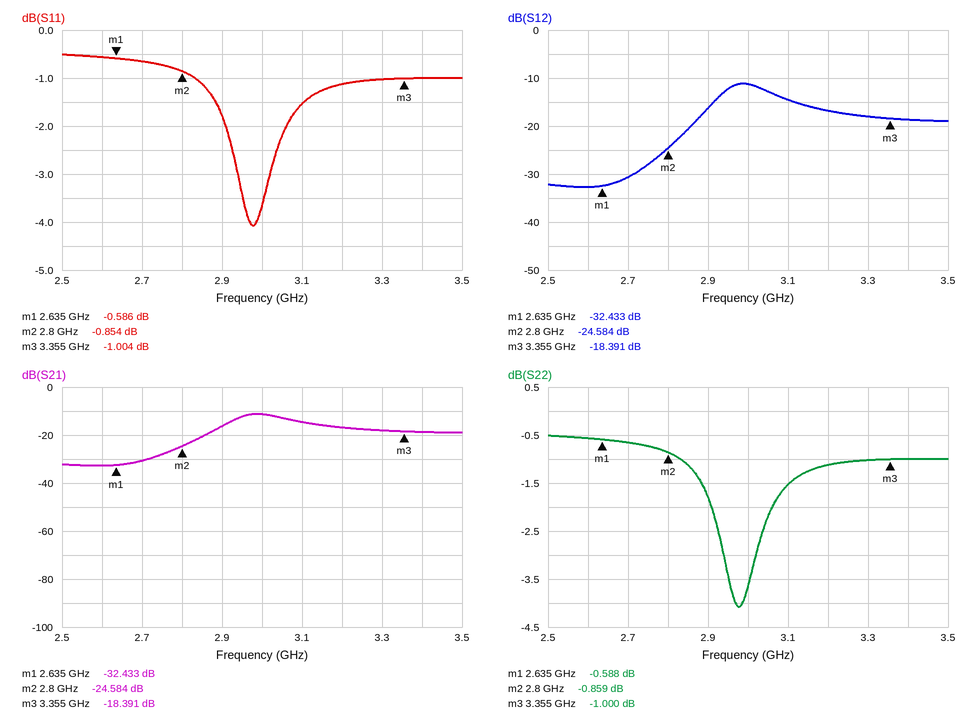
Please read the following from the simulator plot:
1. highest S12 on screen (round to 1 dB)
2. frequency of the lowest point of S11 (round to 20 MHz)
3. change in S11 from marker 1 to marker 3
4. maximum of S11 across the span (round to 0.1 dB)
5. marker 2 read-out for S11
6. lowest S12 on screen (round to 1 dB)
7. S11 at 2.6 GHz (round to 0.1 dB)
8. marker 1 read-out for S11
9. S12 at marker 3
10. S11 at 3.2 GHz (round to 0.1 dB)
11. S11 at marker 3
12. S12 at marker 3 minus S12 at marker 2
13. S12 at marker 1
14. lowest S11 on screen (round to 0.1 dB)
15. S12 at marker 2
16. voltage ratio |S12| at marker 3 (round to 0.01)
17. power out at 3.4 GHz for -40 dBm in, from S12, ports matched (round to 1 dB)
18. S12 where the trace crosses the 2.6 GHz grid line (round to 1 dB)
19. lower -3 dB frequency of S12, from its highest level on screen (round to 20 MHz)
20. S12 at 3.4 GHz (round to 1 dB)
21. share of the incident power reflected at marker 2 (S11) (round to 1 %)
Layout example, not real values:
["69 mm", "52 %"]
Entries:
["-11 dB", "2.98 GHz", "-0.418 dB", "-0.5 dB", "-0.854 dB", "-33 dB", "-0.6 dB", "-0.586 dB", "-18.391 dB", "-1.1 dB", "-1.004 dB", "6.193 dB", "-32.433 dB", "-4.1 dB", "-24.584 dB", "0.12", "-59 dBm", "-33 dB", "2.92 GHz", "-19 dB", "82 %"]
